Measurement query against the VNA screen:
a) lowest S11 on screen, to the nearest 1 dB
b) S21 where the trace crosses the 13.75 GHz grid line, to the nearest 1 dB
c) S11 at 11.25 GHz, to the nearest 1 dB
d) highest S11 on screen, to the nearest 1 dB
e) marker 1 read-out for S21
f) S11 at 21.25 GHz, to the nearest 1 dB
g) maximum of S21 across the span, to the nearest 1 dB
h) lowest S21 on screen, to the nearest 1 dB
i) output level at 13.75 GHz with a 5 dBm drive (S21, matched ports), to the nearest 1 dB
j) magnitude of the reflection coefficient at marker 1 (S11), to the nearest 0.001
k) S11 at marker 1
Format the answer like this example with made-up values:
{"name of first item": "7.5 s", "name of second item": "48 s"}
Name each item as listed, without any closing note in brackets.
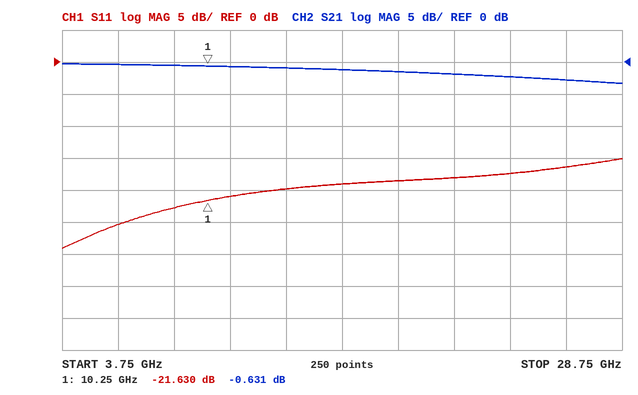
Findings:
{"lowest S11 on screen, to the nearest 1 dB": "-29 dB", "S21 where the trace crosses the 13.75 GHz grid line, to the nearest 1 dB": "-1 dB", "S11 at 11.25 GHz, to the nearest 1 dB": "-21 dB", "highest S11 on screen, to the nearest 1 dB": "-15 dB", "marker 1 read-out for S21": "-0.631 dB", "S11 at 21.25 GHz, to the nearest 1 dB": "-18 dB", "maximum of S21 across the span, to the nearest 1 dB": "0 dB", "lowest S21 on screen, to the nearest 1 dB": "-3 dB", "output level at 13.75 GHz with a 5 dBm drive (S21, matched ports), to the nearest 1 dB": "4 dBm", "magnitude of the reflection coefficient at marker 1 (S11), to the nearest 0.001": "0.083", "S11 at marker 1": "-21.630 dB"}
